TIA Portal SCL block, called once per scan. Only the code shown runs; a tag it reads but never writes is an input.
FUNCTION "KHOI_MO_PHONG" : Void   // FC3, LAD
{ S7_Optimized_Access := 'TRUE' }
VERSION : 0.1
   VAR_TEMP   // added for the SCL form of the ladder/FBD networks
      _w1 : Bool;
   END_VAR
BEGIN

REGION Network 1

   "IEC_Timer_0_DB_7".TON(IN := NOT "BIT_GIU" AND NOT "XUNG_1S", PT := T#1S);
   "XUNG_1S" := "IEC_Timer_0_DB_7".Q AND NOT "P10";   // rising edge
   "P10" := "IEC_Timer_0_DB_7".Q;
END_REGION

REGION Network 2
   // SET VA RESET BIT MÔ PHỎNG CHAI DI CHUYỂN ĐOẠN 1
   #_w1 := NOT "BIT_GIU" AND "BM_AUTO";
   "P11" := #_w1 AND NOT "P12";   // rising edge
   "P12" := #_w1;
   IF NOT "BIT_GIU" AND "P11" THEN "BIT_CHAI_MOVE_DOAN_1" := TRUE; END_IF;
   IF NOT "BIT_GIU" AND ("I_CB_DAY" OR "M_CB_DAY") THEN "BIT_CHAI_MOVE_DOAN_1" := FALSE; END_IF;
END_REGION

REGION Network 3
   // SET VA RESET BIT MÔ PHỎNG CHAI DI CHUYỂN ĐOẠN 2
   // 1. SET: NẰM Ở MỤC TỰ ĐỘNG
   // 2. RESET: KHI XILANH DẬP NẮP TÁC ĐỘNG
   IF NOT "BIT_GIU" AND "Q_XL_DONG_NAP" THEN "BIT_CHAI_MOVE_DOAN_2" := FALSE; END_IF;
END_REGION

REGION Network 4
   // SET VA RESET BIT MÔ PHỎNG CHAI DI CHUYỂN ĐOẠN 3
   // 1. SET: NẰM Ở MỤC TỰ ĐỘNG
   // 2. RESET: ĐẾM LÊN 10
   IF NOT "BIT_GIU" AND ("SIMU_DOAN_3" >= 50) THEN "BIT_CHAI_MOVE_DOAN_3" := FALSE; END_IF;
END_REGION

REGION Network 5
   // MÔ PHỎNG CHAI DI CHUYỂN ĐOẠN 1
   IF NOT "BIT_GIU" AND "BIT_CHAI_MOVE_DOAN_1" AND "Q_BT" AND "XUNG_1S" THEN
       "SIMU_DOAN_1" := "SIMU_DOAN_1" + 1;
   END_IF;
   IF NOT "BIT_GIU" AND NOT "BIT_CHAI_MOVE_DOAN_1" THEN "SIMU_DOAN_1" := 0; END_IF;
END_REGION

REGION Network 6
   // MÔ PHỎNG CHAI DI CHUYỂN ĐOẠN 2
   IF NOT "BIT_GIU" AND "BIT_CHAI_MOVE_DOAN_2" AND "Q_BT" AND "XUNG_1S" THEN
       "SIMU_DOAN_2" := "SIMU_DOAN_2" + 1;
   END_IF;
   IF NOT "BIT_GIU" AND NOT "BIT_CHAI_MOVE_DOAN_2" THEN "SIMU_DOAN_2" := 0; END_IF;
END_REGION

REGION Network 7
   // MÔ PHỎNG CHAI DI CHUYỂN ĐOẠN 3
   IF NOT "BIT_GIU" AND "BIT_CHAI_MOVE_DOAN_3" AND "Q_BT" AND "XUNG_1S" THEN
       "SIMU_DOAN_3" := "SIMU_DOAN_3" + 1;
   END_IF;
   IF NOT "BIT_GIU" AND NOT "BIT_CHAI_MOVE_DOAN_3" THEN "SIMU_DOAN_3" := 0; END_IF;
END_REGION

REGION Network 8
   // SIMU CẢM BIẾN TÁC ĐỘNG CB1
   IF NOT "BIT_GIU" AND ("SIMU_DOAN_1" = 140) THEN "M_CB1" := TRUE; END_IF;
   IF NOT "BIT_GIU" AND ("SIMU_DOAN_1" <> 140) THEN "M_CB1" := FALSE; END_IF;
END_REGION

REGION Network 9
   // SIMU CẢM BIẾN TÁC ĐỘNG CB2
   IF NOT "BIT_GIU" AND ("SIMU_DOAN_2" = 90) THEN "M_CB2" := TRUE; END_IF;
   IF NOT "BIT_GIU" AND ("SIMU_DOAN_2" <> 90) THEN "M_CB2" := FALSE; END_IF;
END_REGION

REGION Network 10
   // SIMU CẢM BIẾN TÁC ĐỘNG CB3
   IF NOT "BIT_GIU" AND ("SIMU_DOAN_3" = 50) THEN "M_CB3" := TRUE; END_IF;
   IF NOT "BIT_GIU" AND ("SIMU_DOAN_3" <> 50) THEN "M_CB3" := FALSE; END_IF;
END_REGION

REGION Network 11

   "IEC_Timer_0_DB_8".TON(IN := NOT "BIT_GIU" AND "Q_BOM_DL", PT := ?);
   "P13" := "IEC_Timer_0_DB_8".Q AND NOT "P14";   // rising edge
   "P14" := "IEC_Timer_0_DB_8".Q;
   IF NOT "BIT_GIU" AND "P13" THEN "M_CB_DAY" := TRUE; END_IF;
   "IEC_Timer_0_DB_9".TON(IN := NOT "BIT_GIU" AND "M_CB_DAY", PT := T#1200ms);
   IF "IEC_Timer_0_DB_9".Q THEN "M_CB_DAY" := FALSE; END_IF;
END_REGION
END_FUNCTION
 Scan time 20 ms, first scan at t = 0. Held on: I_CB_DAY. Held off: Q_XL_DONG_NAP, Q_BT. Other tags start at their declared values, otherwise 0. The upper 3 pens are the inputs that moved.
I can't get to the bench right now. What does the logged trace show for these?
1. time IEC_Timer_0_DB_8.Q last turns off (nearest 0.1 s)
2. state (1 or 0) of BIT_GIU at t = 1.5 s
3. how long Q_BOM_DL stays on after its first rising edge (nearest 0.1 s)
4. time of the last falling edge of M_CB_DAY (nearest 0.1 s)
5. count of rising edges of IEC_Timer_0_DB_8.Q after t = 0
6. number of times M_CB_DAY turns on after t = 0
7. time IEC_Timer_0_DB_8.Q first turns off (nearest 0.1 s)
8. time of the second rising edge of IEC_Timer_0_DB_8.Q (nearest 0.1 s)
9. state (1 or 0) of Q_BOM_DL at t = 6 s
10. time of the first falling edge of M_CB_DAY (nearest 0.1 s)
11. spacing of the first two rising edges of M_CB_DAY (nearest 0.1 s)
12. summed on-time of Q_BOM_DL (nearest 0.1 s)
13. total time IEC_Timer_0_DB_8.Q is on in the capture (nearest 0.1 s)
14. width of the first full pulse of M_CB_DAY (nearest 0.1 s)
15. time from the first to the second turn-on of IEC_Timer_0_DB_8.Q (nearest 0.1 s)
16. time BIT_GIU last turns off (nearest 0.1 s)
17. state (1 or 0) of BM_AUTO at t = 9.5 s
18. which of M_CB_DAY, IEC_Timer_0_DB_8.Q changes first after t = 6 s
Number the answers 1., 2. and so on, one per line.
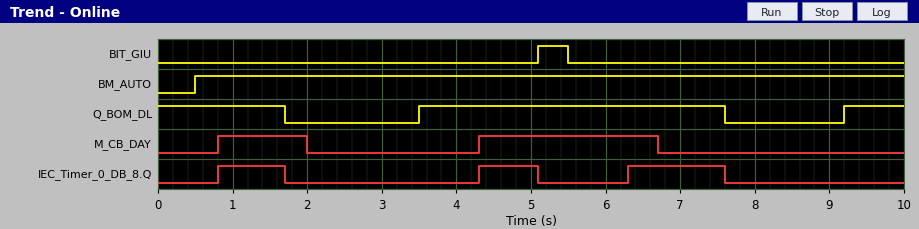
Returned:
1. 7.6 s
2. 0
3. 4.1 s
4. 6.7 s
5. 3
6. 2
7. 1.7 s
8. 4.3 s
9. 1
10. 2.0 s
11. 3.5 s
12. 6.6 s
13. 3.0 s
14. 1.2 s
15. 3.5 s
16. 5.5 s
17. 1
18. IEC_Timer_0_DB_8.Q
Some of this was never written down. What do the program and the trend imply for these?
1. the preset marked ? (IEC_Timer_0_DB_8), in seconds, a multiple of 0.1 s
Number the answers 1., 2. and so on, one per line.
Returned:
1. 0.8 s
